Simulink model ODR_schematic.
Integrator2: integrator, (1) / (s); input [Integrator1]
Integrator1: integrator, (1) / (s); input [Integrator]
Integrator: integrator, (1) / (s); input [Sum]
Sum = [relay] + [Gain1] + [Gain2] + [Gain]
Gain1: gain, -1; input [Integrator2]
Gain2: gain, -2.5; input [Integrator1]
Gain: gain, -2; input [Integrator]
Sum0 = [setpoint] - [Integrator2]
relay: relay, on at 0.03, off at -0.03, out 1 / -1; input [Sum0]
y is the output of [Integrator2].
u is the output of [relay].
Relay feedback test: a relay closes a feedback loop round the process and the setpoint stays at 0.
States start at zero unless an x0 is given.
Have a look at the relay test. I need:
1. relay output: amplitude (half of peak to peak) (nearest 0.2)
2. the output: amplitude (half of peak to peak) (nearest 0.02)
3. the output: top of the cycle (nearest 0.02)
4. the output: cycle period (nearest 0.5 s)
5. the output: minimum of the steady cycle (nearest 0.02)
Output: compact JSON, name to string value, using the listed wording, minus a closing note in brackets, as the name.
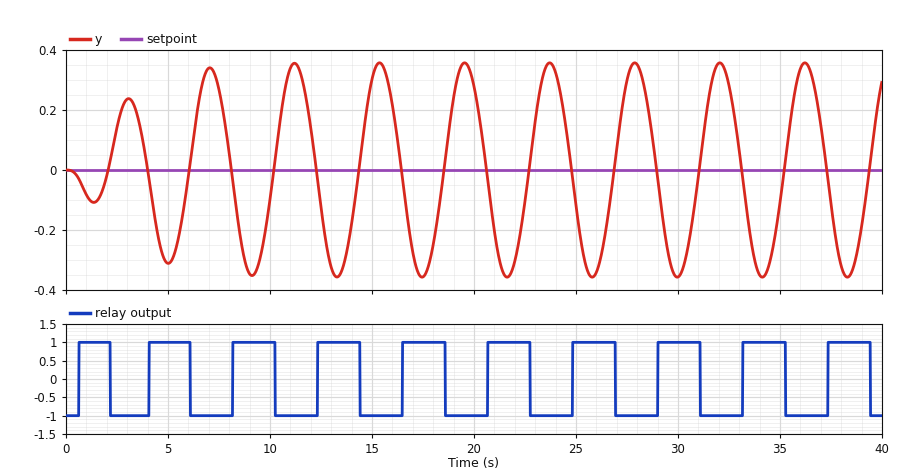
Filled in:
{"relay output: amplitude (half of peak to peak)": "1.0", "the output: amplitude (half of peak to peak)": "0.36", "the output: top of the cycle": "0.36", "the output: cycle period": "4.0 s", "the output: minimum of the steady cycle": "-0.36"}
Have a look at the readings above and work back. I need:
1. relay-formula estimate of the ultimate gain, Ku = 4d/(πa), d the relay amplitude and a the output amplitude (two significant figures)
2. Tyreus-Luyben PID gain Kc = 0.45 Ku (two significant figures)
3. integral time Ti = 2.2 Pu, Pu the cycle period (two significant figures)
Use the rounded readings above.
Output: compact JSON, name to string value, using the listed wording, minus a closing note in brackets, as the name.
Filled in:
{"relay-formula estimate of the ultimate gain, Ku = 4d/(πa), d the relay amplitude and a the output amplitude": "3.5", "Tyreus-Luyben PID gain Kc = 0.45 Ku": "1.6", "integral time Ti = 2.2 Pu, Pu the cycle period": "8.8 s"}
